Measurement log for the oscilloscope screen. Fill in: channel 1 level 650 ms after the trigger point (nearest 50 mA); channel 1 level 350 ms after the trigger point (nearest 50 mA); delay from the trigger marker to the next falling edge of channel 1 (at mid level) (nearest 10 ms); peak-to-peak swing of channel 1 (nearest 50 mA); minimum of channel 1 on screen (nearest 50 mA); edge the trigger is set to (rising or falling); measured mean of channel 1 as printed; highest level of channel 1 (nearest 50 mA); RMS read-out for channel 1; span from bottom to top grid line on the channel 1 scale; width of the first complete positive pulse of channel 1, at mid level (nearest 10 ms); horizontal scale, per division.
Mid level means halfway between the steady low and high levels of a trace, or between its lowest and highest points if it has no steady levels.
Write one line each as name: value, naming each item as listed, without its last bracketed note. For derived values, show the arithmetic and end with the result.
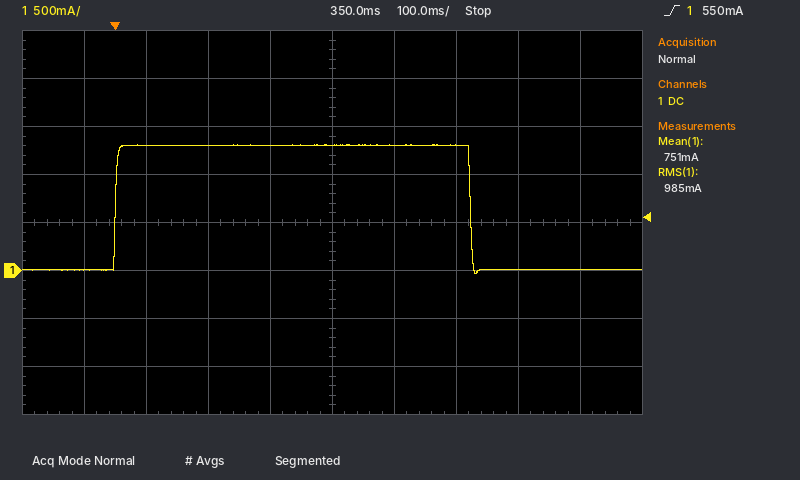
channel 1 level 650 ms after the trigger point: 0 mA
channel 1 level 350 ms after the trigger point: 1.30 A
delay from the trigger marker to the next falling edge of channel 1 (at mid level): 570 ms
peak-to-peak swing of channel 1: 1.30 A − (-50 mA) = 1.35 A
minimum of channel 1 on screen: -50 mA
edge the trigger is set to: rising
measured mean of channel 1 as printed: 751 mA
highest level of channel 1: 1.30 A
RMS read-out for channel 1: 985 mA
span from bottom to top grid line on the channel 1 scale: 4 A
width of the first complete positive pulse of channel 1, at mid level: 570 ms
horizontal scale, per division: 100 ms
